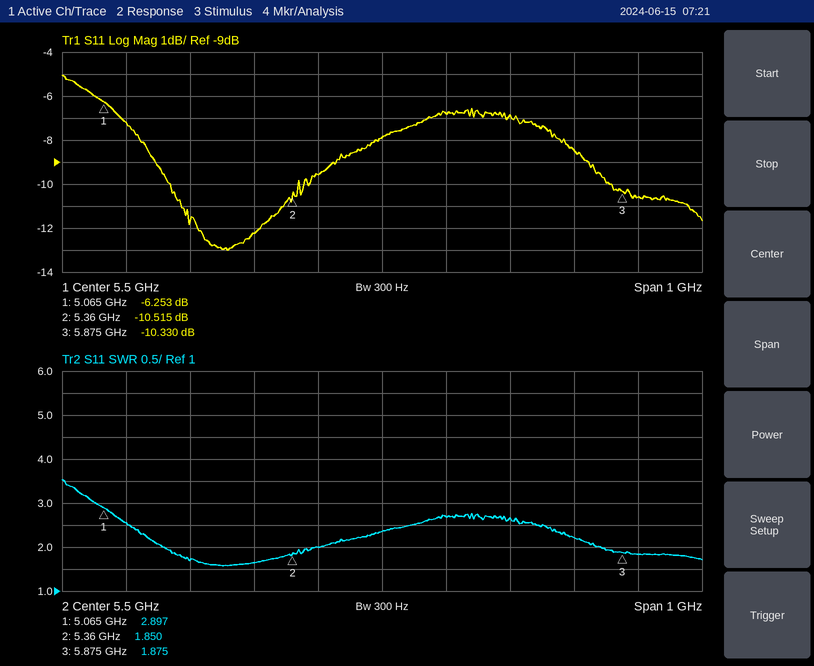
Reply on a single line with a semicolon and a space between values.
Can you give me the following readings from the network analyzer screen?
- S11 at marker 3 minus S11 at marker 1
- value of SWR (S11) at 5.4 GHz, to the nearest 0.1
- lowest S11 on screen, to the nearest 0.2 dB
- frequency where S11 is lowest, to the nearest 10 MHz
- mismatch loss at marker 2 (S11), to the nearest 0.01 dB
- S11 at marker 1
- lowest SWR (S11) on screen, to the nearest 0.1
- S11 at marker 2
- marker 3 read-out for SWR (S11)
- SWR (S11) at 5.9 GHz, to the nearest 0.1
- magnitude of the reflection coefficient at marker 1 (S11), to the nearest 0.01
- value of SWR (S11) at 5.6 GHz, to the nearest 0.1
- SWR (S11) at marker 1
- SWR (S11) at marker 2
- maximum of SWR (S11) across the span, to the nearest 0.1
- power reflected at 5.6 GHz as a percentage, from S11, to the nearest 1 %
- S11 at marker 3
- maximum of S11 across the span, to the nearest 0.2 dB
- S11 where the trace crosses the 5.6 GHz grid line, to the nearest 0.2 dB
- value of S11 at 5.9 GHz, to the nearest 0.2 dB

-4.077 dB; 2.0; -13.0 dB; 5.26 GHz; 0.40 dB; -6.253 dB; 1.6; -10.515 dB; 1.875; 1.8; 0.49; 2.7; 2.897; 1.850; 3.5; 21 %; -10.330 dB; -5.0 dB; -6.8 dB; -10.6 dB
